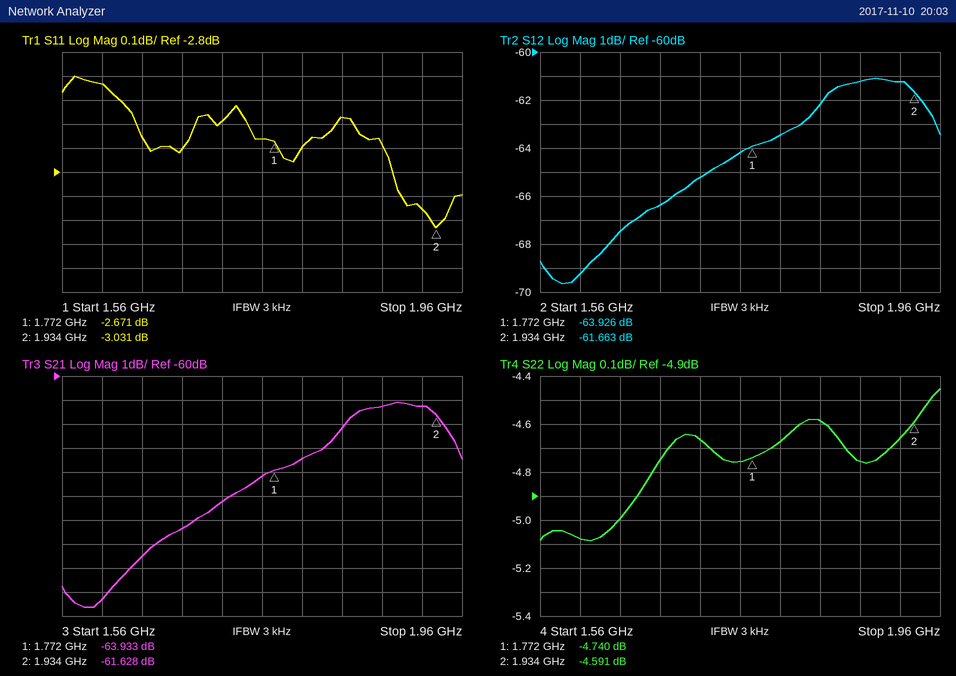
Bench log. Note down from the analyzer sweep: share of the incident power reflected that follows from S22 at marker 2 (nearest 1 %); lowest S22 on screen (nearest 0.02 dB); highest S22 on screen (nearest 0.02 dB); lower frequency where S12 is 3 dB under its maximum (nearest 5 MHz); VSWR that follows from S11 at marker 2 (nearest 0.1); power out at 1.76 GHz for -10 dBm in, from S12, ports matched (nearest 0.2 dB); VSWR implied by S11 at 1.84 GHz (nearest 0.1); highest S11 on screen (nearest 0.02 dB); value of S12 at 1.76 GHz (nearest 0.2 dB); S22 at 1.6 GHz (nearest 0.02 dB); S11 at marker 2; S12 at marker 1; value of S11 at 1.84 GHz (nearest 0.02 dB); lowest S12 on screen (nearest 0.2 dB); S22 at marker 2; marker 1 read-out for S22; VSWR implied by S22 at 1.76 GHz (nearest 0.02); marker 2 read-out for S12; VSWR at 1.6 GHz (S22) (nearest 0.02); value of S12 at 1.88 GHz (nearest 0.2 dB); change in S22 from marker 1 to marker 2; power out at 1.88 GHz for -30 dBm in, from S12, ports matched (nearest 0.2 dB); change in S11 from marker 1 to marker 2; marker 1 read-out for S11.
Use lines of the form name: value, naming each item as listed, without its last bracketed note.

share of the incident power reflected that follows from S22 at marker 2: 35 %
lowest S22 on screen: -5.08 dB
highest S22 on screen: -4.46 dB
lower frequency where S12 is 3 dB under its maximum: 1.765 GHz
VSWR that follows from S11 at marker 2: 5.8
power out at 1.76 GHz for -10 dBm in, from S12, ports matched: -74.2 dBm
VSWR implied by S11 at 1.84 GHz: 6.8
highest S11 on screen: -2.40 dB
value of S12 at 1.76 GHz: -64.2 dB
S22 at 1.6 GHz: -5.08 dB
S11 at marker 2: -3.031 dB
S12 at marker 1: -63.926 dB
value of S11 at 1.84 GHz: -2.58 dB
lowest S12 on screen: -69.6 dB
S22 at marker 2: -4.591 dB
marker 1 read-out for S22: -4.740 dB
VSWR implied by S22 at 1.76 GHz: 3.74
marker 2 read-out for S12: -61.663 dB
VSWR at 1.6 GHz (S22): 3.52
value of S12 at 1.88 GHz: -61.2 dB
change in S22 from marker 1 to marker 2: 0.149 dB
power out at 1.88 GHz for -30 dBm in, from S12, ports matched: -91.2 dBm
change in S11 from marker 1 to marker 2: -0.360 dB
marker 1 read-out for S11: -2.671 dB
